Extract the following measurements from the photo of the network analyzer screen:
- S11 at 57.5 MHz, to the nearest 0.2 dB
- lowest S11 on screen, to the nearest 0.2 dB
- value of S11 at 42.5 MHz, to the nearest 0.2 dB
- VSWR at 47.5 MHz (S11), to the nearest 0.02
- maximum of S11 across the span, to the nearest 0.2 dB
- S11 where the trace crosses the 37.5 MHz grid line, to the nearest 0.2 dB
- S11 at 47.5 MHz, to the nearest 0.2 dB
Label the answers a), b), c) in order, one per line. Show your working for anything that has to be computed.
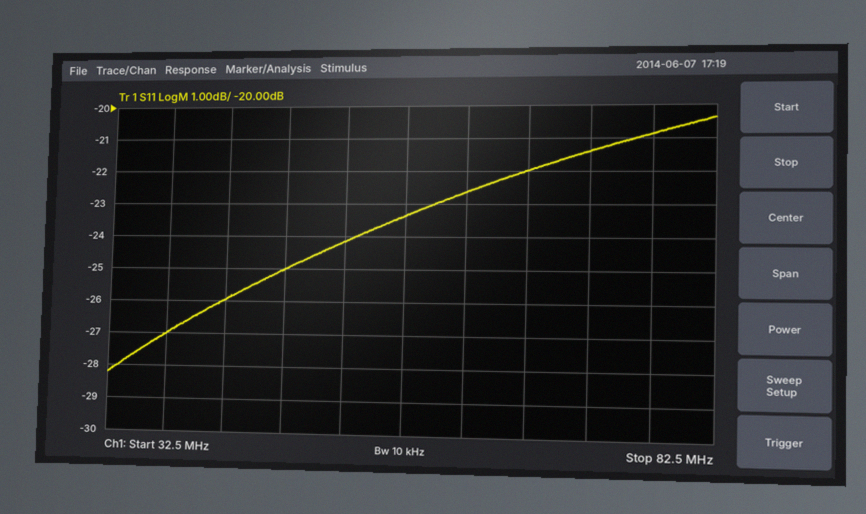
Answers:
a) -23.4 dB
b) -28.2 dB
c) -26.0 dB
d) |Γ| = 10^(-25/20) = 0.0562; VSWR = (1 + 0.0562)/(1 − 0.0562) ≈ 1.12
e) -20.4 dB
f) -27.0 dB
g) -25.0 dB
